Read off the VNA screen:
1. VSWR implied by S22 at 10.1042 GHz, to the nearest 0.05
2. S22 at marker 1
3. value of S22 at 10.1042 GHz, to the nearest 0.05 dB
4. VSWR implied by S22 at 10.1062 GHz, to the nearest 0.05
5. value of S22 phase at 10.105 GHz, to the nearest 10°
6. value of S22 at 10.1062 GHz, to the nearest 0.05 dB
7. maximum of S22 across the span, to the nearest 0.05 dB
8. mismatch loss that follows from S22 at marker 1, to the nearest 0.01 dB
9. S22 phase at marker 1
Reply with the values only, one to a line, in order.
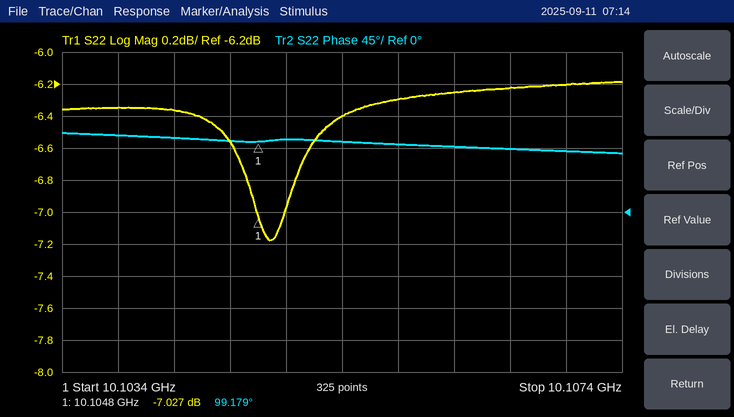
2.85
-7.027 dB
-6.35 dB
2.90
100°
-6.25 dB
-6.20 dB
0.96 dB
99.179°
